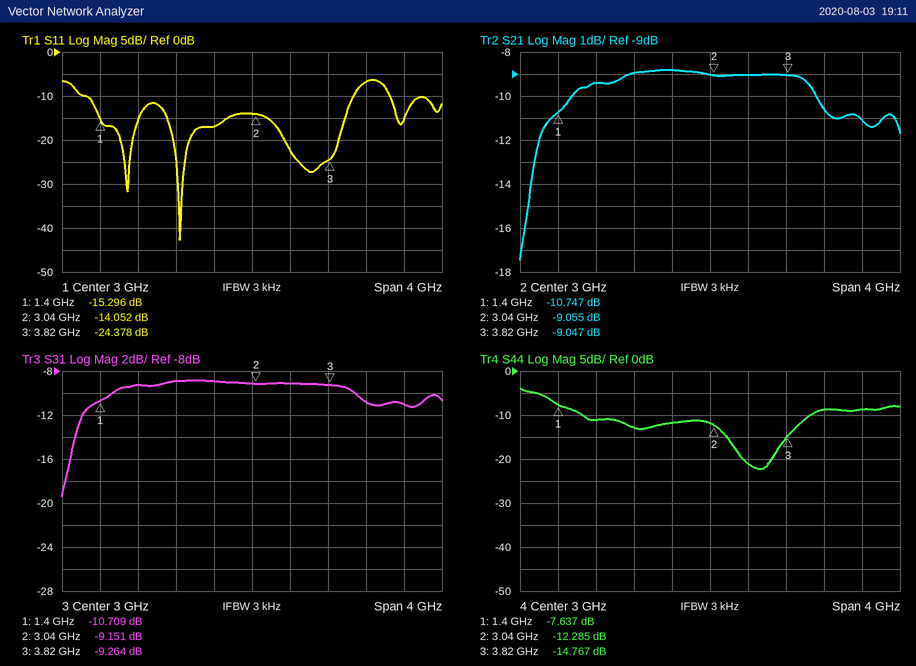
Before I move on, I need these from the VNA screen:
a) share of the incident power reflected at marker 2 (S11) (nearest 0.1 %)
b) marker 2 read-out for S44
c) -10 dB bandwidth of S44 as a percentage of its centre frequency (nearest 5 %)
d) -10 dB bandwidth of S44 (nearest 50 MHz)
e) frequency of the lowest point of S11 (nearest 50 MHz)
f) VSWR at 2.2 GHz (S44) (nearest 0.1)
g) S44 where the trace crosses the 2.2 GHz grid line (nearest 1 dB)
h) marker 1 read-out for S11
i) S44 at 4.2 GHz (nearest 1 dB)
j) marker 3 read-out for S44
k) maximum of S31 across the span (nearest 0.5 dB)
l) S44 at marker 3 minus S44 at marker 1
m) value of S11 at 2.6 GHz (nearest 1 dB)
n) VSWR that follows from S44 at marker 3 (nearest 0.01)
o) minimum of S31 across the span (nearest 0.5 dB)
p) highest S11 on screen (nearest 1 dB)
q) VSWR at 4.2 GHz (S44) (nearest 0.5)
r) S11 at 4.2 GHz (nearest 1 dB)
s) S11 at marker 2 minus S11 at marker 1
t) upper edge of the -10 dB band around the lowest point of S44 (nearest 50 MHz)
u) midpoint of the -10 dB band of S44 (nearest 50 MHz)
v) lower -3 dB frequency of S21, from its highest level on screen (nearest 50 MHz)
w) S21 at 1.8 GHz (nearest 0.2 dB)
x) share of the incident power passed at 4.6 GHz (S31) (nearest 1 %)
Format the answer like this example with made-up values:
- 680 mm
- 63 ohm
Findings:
- 3.9 %
- -12.285 dB
- 85 %
- 2.40 GHz
- 2.25 GHz
- 1.6
- -13 dB
- -15.296 dB
- -9 dB
- -14.767 dB
- -9.0 dB
- -7.130 dB
- -17 dB
- 1.45
- -19.5 dB
- -6 dB
- 2.0
- -7 dB
- 1.244 dB
- 4.05 GHz
- 2.85 GHz
- 1.20 GHz
- -9.4 dB
- 8 %
